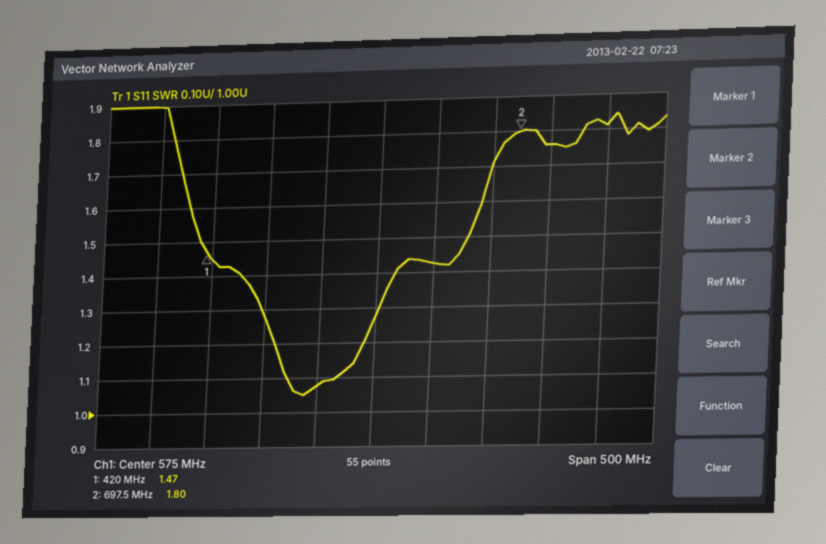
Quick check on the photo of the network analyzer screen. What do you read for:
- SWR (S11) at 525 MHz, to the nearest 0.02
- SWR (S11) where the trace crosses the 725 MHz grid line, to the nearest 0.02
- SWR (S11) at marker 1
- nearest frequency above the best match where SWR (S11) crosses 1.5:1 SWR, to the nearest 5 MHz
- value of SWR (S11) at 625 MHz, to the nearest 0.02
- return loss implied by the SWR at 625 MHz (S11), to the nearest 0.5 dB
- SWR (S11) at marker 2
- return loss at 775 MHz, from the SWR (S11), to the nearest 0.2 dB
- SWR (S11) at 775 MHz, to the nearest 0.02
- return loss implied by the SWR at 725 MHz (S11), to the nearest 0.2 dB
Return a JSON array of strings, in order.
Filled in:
["1.08", "1.76", "1.47", "655 MHz", "1.42", "15.0 dB", "1.80", "10.8 dB", "1.82", "11.2 dB"]
